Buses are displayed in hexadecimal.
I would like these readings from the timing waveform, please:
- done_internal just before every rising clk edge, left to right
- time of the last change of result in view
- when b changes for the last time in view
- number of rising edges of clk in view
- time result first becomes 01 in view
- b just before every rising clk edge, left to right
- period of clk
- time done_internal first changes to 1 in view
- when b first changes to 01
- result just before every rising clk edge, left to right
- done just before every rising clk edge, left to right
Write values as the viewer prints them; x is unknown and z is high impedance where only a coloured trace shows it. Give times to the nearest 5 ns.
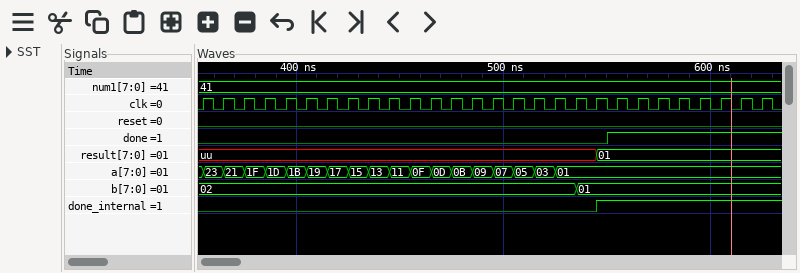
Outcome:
0 0 0 0 0 0 0 0 0 0 0 0 0 0 0 0 0 0 0 0 1 1 1 1 1 1 1 1
545 ns
535 ns
28
545 ns
02, 02, 02, 02, 02, 02, 02, 02, 02, 02, 02, 02, 02, 02, 02, 02, 02, 02, 02, 01, 01, 01, 01, 01, 01, 01, 01, 01
10 ns
545 ns
535 ns
uu, uu, uu, uu, uu, uu, uu, uu, uu, uu, uu, uu, uu, uu, uu, uu, uu, uu, uu, uu, 01, 01, 01, 01, 01, 01, 01, 01
0 0 0 0 0 0 0 0 0 0 0 0 0 0 0 0 0 0 0 0 1 1 1 1 1 1 1 1
